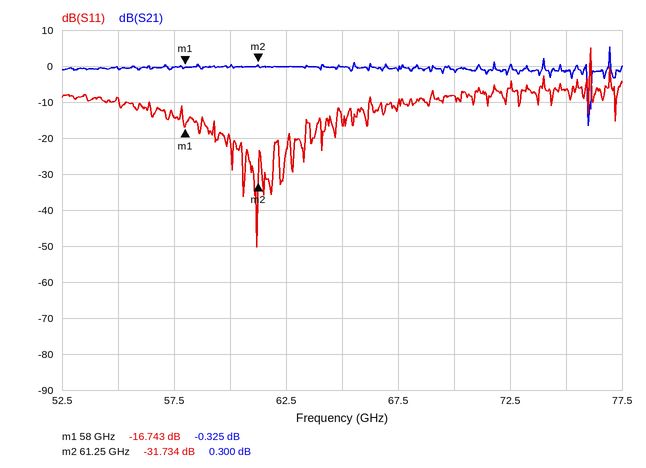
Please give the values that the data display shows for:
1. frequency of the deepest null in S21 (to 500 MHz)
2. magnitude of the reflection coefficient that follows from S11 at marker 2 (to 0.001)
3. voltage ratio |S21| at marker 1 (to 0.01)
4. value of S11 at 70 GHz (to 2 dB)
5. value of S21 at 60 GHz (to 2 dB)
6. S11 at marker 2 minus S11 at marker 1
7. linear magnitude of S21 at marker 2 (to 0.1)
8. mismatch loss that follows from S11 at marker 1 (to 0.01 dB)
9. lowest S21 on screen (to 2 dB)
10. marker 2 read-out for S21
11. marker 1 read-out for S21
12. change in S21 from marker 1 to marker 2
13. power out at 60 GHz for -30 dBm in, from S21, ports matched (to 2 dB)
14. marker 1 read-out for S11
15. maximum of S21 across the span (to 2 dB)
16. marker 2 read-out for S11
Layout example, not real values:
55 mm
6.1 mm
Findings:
76.0 GHz
0.026
0.96
-8 dB
0 dB
-14.991 dB
1.0
0.09 dB
-16 dB
0.300 dB
-0.325 dB
0.625 dB
-30 dBm
-16.743 dB
6 dB
-31.734 dB
